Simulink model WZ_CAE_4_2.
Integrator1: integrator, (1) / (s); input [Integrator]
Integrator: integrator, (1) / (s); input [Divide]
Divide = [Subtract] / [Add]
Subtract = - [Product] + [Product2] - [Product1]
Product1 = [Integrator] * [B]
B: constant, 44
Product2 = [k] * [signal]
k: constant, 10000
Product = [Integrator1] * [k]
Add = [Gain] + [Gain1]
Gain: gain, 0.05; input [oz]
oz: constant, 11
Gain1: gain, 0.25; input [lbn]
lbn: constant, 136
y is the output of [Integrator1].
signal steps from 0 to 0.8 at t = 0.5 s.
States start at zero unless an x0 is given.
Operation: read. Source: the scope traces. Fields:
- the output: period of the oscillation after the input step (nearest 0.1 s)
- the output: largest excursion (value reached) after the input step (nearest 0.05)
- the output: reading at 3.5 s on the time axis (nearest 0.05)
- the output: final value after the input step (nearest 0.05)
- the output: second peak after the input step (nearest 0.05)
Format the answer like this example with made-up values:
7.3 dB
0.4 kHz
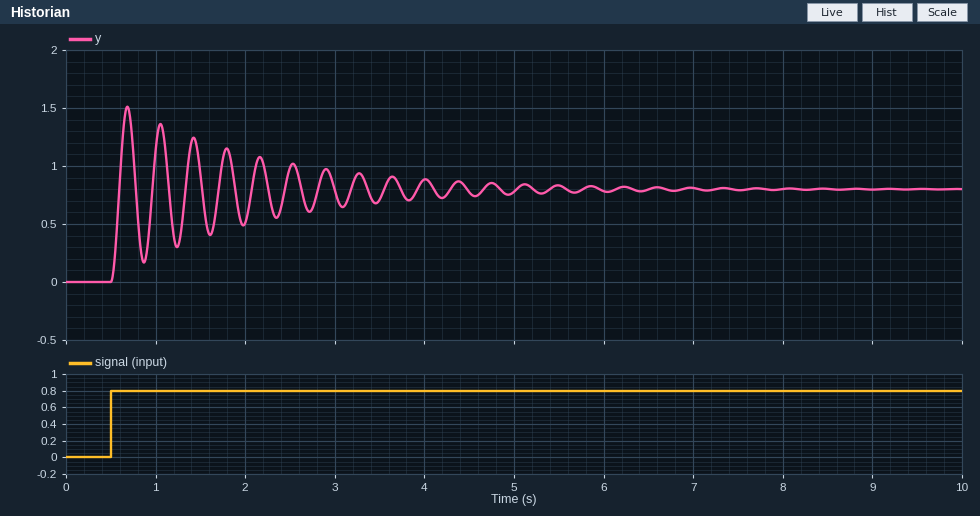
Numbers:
0.4 s
1.50
0.70
0.80
1.35
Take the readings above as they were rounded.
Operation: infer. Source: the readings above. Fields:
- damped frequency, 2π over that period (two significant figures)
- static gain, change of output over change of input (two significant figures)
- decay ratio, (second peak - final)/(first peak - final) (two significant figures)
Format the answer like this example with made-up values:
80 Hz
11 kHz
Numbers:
16 rad/s
1.0
0.79
